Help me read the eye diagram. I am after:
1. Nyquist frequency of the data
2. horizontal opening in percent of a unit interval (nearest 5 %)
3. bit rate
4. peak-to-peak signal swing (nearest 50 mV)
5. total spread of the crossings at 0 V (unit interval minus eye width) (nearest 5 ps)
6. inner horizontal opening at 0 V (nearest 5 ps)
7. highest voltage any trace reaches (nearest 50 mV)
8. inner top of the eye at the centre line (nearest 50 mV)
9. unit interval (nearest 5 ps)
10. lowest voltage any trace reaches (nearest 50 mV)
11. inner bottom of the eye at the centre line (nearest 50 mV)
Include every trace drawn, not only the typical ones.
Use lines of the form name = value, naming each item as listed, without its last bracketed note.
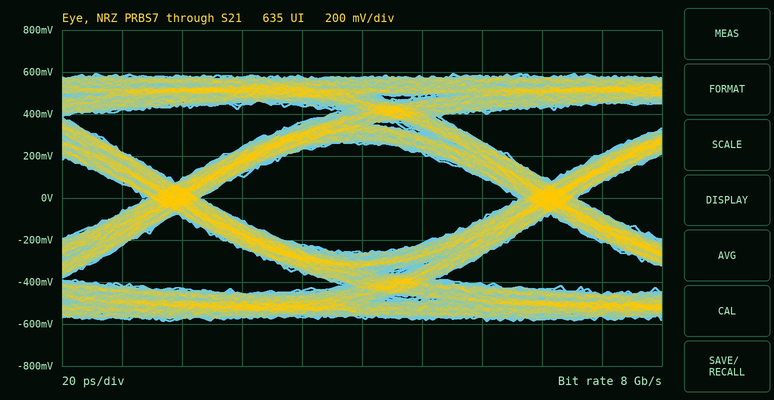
Nyquist frequency of the data = 4 GHz
horizontal opening in percent of a unit interval = 85 %
bit rate = 8 Gb/s
peak-to-peak signal swing = 1.20 V
total spread of the crossings at 0 V (unit interval minus eye width) = 20 ps
inner horizontal opening at 0 V = 105 ps
highest voltage any trace reaches = 600 mV
inner top of the eye at the centre line = 250 mV
unit interval = 125 ps
lowest voltage any trace reaches = -600 mV
inner bottom of the eye at the centre line = -250 mV
